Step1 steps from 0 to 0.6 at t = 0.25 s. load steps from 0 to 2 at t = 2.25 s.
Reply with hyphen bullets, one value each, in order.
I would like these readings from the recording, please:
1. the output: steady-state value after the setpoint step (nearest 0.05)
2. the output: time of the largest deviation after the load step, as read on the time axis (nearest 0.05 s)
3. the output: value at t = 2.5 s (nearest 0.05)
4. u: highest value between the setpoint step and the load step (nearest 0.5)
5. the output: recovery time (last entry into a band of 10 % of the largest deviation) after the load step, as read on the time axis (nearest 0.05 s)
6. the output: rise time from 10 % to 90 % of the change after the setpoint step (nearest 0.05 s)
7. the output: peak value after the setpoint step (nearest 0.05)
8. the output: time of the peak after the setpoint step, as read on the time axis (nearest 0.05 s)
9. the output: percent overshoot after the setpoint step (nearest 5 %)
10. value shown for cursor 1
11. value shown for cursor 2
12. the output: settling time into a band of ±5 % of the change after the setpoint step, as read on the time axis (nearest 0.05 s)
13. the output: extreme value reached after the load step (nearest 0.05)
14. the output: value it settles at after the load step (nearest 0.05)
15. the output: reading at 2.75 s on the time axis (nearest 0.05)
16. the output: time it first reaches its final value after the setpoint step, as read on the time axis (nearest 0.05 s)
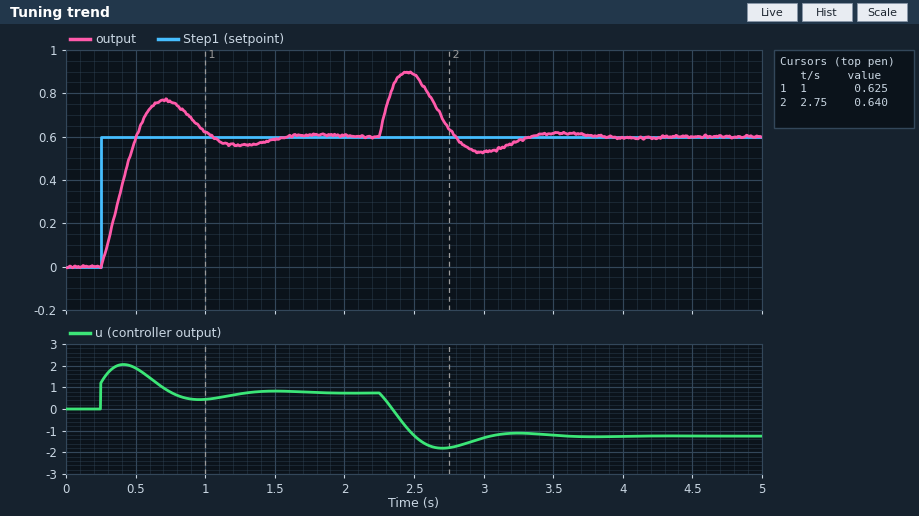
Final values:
- 0.60
- 2.45 s
- 0.90
- 2.0
- 3.20 s
- 0.20 s
- 0.75
- 0.70 s
- 30 %
- 0.625
- 0.640
- 1.40 s
- 0.90
- 0.60
- 0.65
- 0.50 s
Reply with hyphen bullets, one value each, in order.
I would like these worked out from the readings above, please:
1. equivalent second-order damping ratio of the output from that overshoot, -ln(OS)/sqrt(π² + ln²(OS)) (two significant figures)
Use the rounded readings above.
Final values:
- 0.36
